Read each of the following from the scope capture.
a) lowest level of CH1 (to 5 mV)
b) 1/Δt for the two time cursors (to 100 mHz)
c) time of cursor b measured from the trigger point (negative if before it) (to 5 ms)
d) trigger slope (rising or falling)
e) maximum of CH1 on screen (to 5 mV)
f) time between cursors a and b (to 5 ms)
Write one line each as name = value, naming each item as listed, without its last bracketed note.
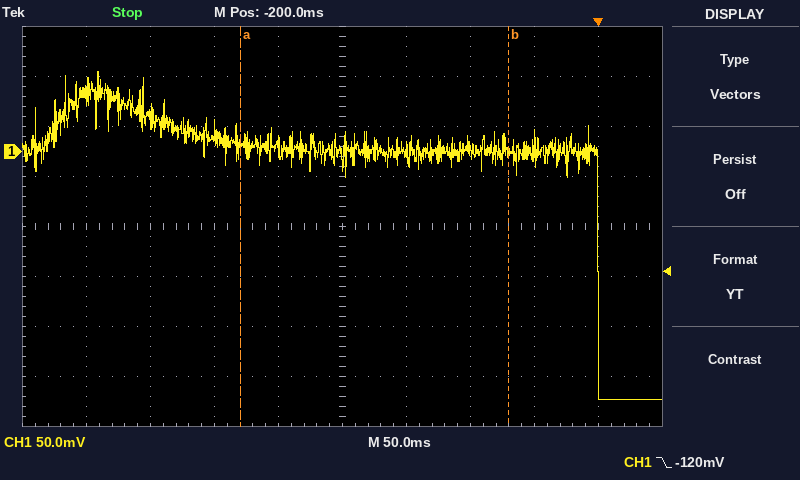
lowest level of CH1 = -250 mV
1/Δt for the two time cursors = 4.8 Hz
time of cursor b measured from the trigger point (negative if before it) = -70 ms
trigger slope = falling
maximum of CH1 on screen = 80 mV
time between cursors a and b = 210 ms
